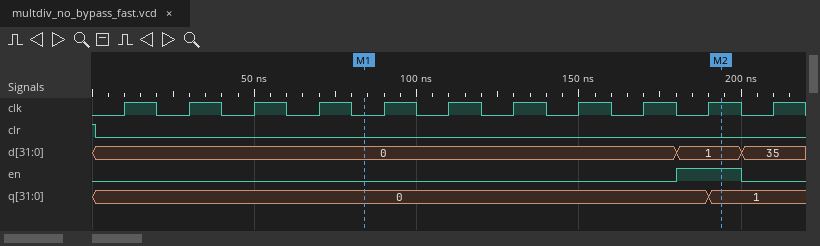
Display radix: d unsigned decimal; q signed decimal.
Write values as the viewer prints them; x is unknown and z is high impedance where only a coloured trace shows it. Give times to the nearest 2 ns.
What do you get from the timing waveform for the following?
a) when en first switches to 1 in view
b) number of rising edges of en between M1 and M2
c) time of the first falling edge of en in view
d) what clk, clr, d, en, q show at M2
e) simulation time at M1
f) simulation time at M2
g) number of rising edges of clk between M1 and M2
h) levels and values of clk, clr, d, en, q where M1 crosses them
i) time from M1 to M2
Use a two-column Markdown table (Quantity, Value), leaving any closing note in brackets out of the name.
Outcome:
| Quantity | Value |
|---|---|
| when en first switches to 1 in view | 180 ns |
| number of rising edges of en between M1 and M2 | 1 |
| time of the first falling edge of en in view | 200 ns |
| what clk, clr, d, en, q show at M2 | clk=1, clr=0, d=1, en=1, q=1 |
| simulation time at M1 | 84 ns |
| simulation time at M2 | 194 ns |
| number of rising edges of clk between M1 and M2 | 6 |
| levels and values of clk, clr, d, en, q where M1 crosses them | clk=0, clr=0, d=0, en=0, q=0 |
| time from M1 to M2 | 110 ns |
